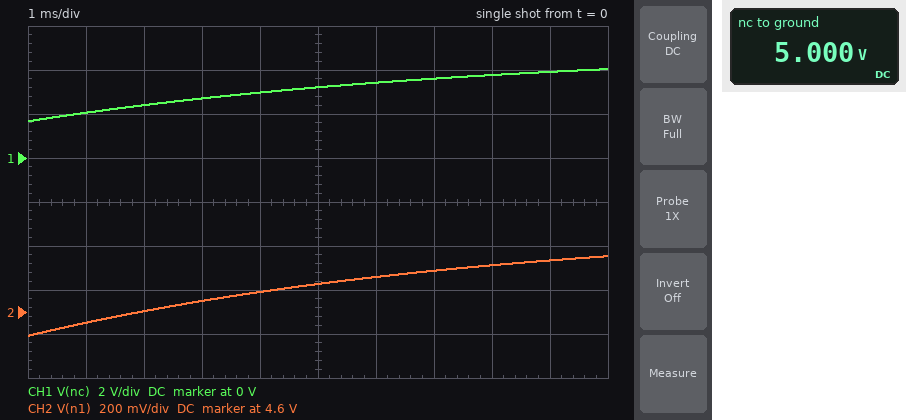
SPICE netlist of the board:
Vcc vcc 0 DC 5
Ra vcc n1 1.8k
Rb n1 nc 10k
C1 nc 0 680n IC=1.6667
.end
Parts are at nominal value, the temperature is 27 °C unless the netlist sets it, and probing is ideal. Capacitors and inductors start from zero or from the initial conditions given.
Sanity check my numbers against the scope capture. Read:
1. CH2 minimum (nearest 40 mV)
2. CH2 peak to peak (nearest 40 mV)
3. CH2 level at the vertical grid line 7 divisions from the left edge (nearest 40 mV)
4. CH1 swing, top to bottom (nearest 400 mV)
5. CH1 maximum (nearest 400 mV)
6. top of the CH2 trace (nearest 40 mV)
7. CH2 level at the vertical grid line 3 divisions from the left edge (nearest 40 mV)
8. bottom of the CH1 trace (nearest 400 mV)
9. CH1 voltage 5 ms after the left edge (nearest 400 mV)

4.48 V
360 mV
4.80 V
2.4 V
4.0 V
4.84 V
4.64 V
1.6 V
3.2 V
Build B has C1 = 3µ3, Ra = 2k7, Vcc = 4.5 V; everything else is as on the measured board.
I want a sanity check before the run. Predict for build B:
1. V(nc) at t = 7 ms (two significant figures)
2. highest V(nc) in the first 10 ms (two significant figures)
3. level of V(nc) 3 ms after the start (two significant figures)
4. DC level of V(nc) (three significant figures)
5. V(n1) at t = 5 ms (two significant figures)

2.1 V
2.3 V
1.9 V
4.50 V
4.0 V
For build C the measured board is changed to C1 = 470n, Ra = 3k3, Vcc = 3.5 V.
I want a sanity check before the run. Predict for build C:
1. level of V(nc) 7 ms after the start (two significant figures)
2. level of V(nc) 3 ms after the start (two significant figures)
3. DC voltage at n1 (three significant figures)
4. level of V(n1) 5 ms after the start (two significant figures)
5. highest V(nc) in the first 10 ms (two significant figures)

2.9 V
2.4 V
3.50 V
3.3 V
3.1 V
